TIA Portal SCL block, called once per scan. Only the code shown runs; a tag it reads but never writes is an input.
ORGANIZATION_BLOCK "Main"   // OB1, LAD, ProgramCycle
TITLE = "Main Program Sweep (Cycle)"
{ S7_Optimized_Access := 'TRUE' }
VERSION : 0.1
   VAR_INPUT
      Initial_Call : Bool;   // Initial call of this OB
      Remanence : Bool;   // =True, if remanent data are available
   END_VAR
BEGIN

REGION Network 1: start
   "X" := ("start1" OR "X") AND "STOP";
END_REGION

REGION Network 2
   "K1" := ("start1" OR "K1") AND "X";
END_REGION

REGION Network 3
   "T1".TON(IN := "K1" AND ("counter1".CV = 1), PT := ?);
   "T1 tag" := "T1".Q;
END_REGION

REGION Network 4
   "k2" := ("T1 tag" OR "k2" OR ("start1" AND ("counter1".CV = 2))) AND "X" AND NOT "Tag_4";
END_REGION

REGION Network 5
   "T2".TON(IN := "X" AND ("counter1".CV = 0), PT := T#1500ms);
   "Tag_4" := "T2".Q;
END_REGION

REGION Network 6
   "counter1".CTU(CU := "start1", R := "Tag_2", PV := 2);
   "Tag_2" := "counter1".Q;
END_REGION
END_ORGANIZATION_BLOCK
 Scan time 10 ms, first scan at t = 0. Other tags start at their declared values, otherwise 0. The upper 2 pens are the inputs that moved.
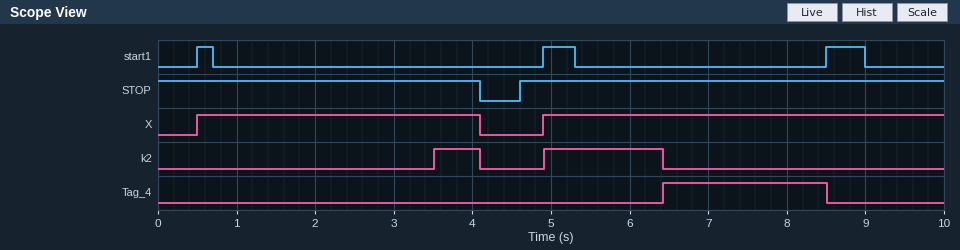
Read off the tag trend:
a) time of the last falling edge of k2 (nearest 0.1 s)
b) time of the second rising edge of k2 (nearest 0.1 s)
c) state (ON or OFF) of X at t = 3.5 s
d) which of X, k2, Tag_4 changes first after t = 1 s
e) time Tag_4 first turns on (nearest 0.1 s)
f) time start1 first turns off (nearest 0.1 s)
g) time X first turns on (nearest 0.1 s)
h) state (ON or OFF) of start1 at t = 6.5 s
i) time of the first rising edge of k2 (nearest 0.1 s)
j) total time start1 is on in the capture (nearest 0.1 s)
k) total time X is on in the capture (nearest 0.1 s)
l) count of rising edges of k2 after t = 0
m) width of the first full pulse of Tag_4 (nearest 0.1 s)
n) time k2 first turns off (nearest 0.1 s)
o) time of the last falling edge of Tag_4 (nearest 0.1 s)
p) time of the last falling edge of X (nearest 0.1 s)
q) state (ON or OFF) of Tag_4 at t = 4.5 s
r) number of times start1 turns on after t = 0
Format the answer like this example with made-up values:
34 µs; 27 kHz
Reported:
6.4 s; 4.9 s; ON; k2; 6.4 s; 0.7 s; 0.5 s; OFF; 3.5 s; 1.1 s; 8.7 s; 2; 2.1 s; 4.1 s; 8.5 s; 4.1 s; OFF; 3
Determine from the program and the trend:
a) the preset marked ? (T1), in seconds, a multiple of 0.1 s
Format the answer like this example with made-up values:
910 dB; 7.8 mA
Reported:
3.0 s
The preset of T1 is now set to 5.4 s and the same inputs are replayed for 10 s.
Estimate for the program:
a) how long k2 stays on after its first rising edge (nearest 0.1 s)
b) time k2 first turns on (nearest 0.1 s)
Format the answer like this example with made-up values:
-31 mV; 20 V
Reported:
1.5 s; 4.9 s
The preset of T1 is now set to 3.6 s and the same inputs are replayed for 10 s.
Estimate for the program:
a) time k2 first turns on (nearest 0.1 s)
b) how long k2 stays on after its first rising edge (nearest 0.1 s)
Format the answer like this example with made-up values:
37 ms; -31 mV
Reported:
4.9 s; 1.5 s
